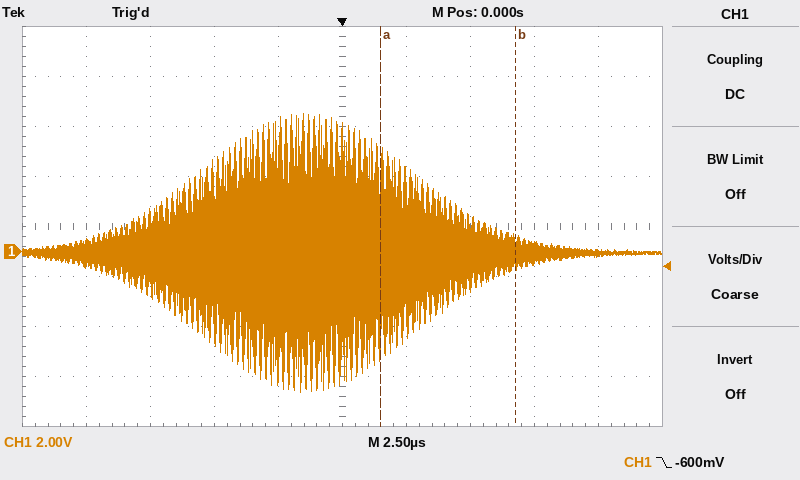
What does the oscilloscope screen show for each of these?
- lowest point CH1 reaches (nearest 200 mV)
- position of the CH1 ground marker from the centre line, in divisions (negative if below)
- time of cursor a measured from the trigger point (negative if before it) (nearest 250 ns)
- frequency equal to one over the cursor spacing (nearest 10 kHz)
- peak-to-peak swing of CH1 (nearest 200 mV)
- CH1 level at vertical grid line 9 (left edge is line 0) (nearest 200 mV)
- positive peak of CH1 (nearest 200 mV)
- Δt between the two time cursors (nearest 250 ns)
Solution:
-5.6 V
-0.5 div
+1.50 µs
190 kHz
11.2 V
0.0 V
5.6 V
5.25 µs
